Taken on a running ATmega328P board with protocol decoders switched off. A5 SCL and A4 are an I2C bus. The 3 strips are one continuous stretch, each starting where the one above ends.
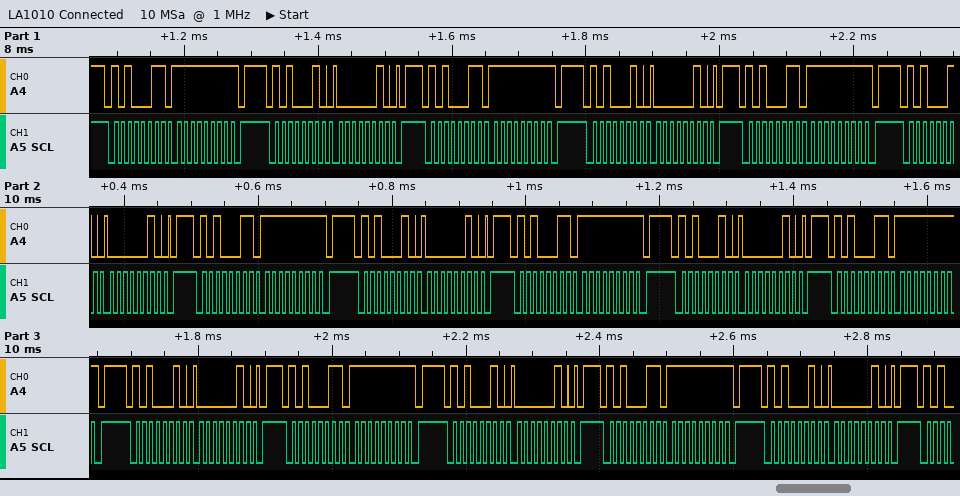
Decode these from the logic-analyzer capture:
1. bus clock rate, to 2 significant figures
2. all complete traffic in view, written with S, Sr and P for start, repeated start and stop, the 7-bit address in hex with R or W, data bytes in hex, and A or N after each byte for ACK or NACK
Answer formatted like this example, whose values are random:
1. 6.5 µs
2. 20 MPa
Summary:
1. 100 kHz
2. S 51R A FF N P S 51W A 02 A P S 51R A FF N P S 51W A 02 A P S 51R A FF N P S 51W A 02 A P S 51R A FF N P S 51W A 02 A P S 51R A FF N P S 51W A 02 A P S 51R A FF N P S 51W A 02 A P S 51R A FF N P S 51W A 02 A P S 51R A FF N P S 51W A 02 A P
